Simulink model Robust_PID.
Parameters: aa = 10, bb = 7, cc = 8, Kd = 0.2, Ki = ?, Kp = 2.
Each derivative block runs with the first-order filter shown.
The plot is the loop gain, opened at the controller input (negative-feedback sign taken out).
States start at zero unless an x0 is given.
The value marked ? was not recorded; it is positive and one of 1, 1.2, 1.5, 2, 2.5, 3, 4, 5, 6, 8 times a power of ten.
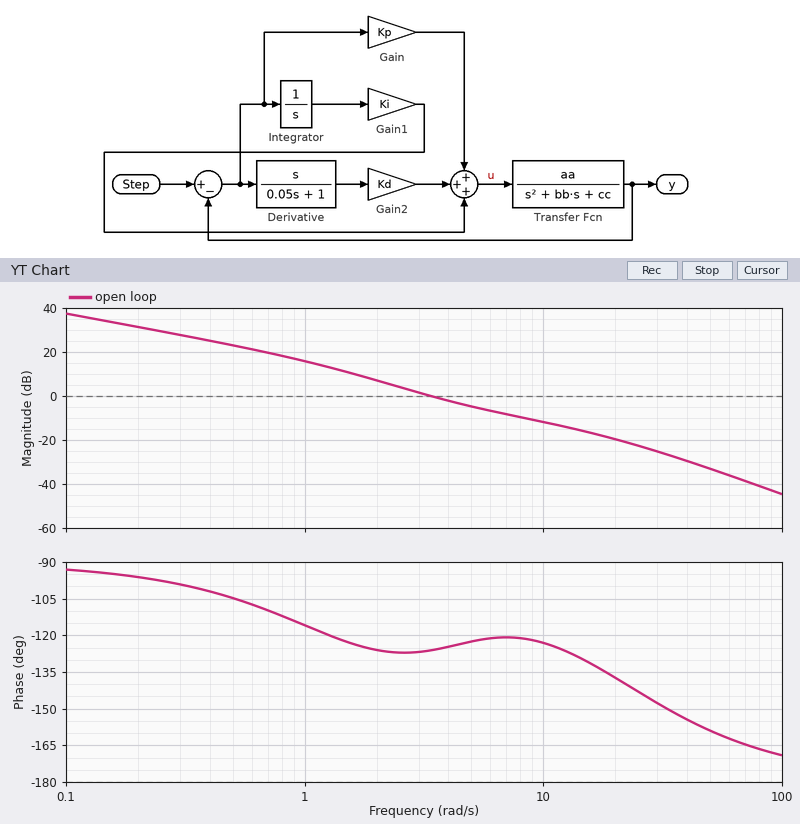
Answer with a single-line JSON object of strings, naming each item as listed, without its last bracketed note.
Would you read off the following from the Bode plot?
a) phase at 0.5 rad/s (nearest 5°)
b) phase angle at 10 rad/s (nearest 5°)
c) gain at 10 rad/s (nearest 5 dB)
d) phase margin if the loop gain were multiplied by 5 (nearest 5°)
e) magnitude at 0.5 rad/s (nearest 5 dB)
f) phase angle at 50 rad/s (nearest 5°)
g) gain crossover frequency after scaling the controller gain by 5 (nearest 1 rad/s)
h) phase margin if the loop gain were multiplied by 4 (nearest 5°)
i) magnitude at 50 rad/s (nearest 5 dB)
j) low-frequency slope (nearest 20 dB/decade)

{"phase at 0.5 rad/s": "-105°", "phase angle at 10 rad/s": "-125°", "gain at 10 rad/s": "-10 dB", "phase margin if the loop gain were multiplied by 5": "55°", "magnitude at 0.5 rad/s": "25 dB", "phase angle at 50 rad/s": "-160°", "gain crossover frequency after scaling the controller gain by 5": "12 rad/s", "phase margin if the loop gain were multiplied by 4": "55°", "magnitude at 50 rad/s": "-35 dB", "low-frequency slope": "-20 dB/decade"}
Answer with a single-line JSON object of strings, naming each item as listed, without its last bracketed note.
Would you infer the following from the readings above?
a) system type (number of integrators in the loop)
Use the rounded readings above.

{"system type": "1"}
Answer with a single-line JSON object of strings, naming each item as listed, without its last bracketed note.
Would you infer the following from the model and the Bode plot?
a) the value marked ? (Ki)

{"the value marked ?": "6"}
